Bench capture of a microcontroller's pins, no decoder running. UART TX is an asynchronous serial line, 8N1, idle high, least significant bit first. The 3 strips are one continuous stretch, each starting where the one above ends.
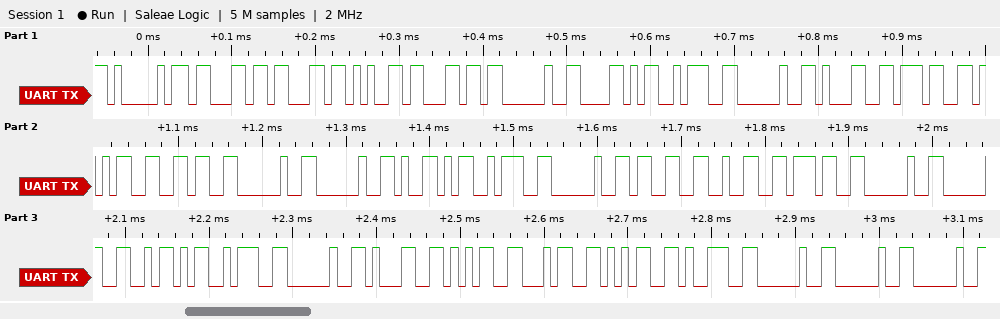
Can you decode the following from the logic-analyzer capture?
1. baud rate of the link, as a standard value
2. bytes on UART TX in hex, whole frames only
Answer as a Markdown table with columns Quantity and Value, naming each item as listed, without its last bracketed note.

| Quantity | Value |
|---|---|
| baud rate of the link, as a standard value | 115200 baud |
| bytes on UART TX in hex, whole frames only | 41 63 63 65 6C 20 58 3A 20 31 37 35 36 20 20 59 3A 20 33 32 37 20 20 5A 3A 20 31 35 34 35 39 20 20 20 |
